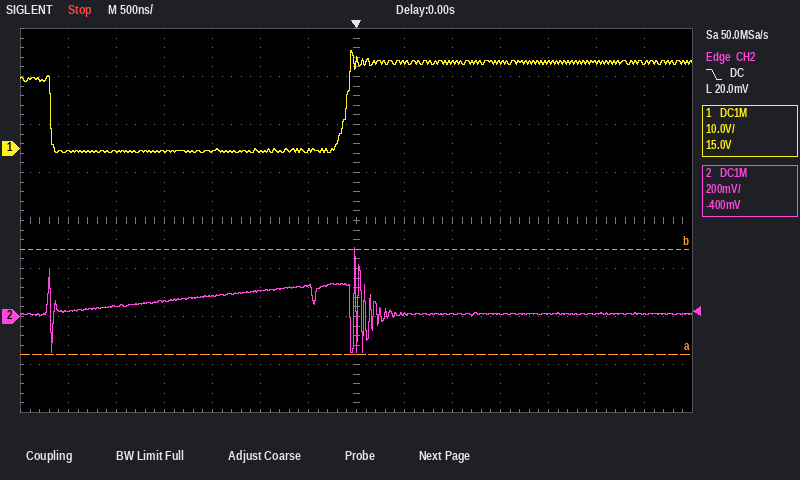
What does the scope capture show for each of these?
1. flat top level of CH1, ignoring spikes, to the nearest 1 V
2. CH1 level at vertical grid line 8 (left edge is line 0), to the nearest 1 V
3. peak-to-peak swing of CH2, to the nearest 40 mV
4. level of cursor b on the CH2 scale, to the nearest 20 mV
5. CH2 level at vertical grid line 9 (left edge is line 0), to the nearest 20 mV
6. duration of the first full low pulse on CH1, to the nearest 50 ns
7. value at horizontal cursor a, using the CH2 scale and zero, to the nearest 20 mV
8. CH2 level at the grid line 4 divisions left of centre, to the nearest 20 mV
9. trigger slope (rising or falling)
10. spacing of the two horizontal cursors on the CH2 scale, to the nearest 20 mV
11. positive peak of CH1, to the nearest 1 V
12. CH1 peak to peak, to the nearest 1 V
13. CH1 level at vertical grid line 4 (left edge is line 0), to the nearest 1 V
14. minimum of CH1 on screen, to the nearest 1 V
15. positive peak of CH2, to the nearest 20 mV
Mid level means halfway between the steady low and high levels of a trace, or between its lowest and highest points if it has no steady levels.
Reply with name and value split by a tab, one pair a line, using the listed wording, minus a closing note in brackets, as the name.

flat top level of CH1, ignoring spikes, to the nearest 1 V	18 V
CH1 level at vertical grid line 8 (left edge is line 0), to the nearest 1 V	18 V
peak-to-peak swing of CH2, to the nearest 40 mV	440 mV
level of cursor b on the CH2 scale, to the nearest 20 mV	280 mV
CH2 level at vertical grid line 9 (left edge is line 0), to the nearest 20 mV	20 mV
duration of the first full low pulse on CH1, to the nearest 50 ns	3.10 µs
value at horizontal cursor a, using the CH2 scale and zero, to the nearest 20 mV	-160 mV
CH2 level at the grid line 4 divisions left of centre, to the nearest 20 mV	60 mV
trigger slope	falling
spacing of the two horizontal cursors on the CH2 scale, to the nearest 20 mV	440 mV
positive peak of CH1, to the nearest 1 V	20 V
CH1 peak to peak, to the nearest 1 V	21 V
CH1 level at vertical grid line 4 (left edge is line 0), to the nearest 1 V	-1 V
minimum of CH1 on screen, to the nearest 1 V	-1 V
positive peak of CH2, to the nearest 20 mV	280 mV
